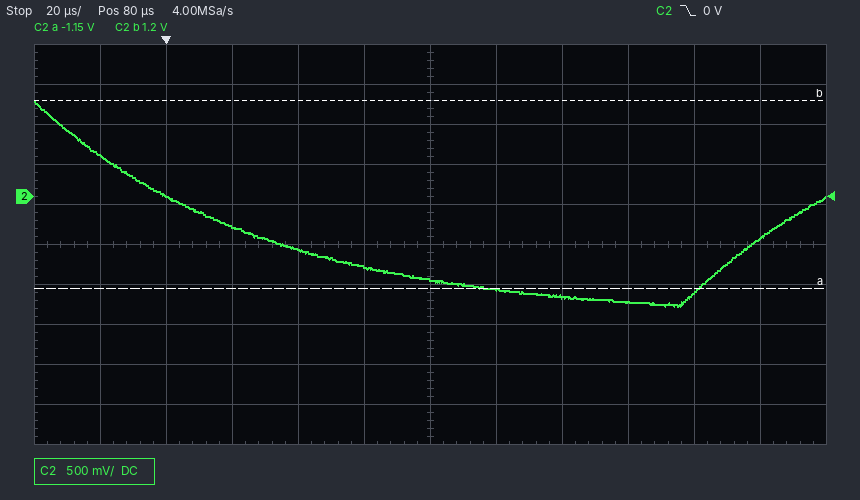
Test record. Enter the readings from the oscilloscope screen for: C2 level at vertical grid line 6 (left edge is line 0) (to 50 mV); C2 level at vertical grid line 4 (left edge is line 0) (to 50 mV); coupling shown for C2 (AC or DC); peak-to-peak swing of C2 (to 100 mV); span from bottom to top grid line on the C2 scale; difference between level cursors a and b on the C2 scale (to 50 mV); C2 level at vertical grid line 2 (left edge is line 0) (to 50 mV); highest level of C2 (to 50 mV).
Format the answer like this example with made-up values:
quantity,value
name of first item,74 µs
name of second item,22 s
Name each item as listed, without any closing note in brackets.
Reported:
quantity,value
C2 level at vertical grid line 6 (left edge is line 0),-1.05 V
C2 level at vertical grid line 4 (left edge is line 0),-650 mV
coupling shown for C2,DC
peak-to-peak swing of C2,2.60 V
span from bottom to top grid line on the C2 scale,5 V
difference between level cursors a and b on the C2 scale,2.35 V
C2 level at vertical grid line 2 (left edge is line 0),0 mV
highest level of C2,1.20 V
